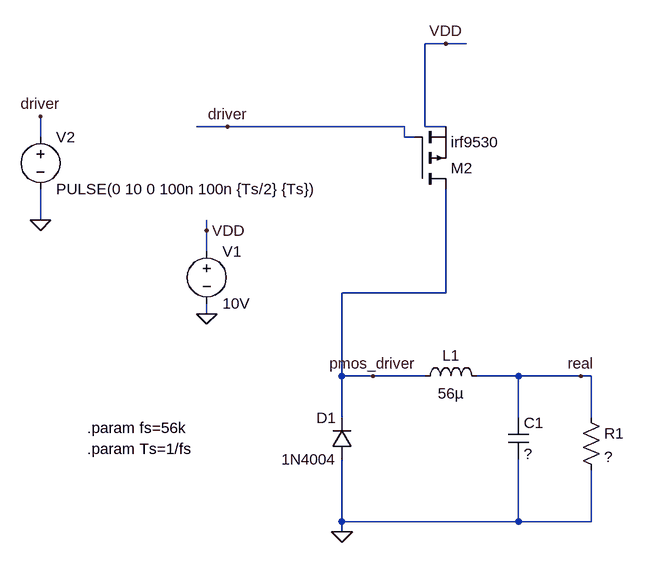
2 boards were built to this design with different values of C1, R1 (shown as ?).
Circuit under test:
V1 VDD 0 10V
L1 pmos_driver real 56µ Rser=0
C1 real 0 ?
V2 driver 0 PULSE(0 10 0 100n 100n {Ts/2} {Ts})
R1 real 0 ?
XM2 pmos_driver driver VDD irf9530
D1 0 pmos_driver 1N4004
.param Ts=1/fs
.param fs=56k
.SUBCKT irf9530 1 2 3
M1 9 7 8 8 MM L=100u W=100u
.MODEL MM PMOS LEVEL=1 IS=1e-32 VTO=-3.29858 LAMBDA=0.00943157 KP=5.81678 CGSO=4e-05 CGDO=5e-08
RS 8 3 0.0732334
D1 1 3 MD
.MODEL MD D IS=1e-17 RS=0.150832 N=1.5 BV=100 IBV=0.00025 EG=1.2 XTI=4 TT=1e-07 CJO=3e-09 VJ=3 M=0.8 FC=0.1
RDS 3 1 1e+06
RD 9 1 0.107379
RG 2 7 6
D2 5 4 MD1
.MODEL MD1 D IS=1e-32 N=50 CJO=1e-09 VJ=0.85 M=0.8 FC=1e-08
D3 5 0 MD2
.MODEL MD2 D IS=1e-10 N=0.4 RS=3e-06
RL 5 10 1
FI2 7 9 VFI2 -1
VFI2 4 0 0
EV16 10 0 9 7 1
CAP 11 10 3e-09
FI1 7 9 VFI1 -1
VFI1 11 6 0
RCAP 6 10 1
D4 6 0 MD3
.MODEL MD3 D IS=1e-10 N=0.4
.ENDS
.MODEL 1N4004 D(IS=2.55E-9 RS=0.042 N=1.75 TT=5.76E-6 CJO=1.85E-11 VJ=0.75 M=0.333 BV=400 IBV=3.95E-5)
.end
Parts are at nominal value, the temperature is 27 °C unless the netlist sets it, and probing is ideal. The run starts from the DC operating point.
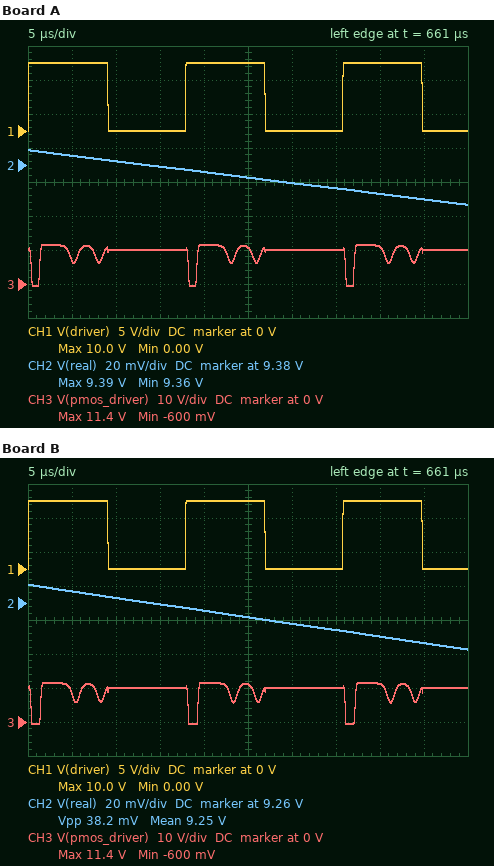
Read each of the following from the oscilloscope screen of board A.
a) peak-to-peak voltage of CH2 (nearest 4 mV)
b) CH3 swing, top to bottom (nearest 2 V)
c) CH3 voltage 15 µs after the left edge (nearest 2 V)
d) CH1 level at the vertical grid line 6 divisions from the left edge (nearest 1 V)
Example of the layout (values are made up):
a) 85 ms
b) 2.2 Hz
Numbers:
a) 32 mV
b) 12 V
c) 10 V
d) 0 V
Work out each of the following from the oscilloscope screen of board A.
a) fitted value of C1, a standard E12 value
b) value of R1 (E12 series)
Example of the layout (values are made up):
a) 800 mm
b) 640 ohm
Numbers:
a) 1.2 mF
b) 12 Ω
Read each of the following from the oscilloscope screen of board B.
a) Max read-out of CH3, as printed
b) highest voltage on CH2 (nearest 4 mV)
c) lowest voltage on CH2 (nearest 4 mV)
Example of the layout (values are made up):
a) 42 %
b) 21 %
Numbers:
a) 11.4 V
b) 9.272 V
c) 9.232 V
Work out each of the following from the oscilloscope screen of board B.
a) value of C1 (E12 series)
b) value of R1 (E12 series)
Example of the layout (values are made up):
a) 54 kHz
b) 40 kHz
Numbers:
a) 1.2 mF
b) 10 Ω
